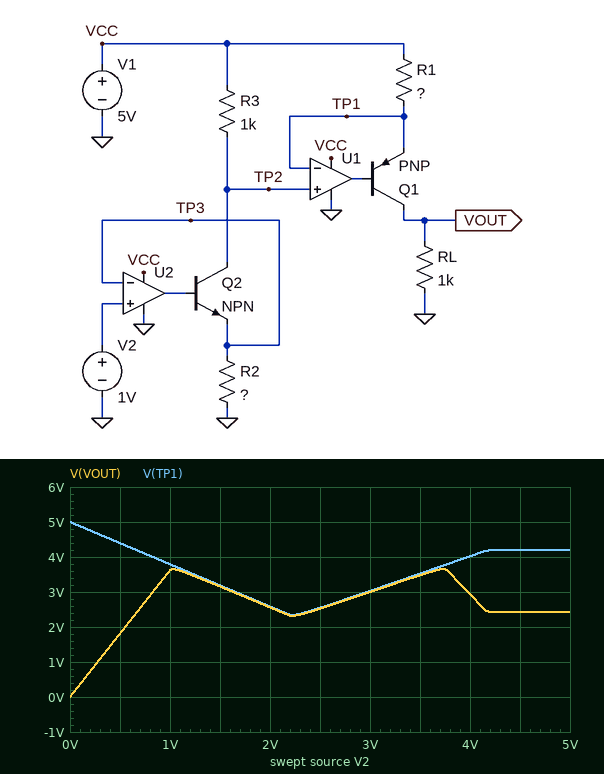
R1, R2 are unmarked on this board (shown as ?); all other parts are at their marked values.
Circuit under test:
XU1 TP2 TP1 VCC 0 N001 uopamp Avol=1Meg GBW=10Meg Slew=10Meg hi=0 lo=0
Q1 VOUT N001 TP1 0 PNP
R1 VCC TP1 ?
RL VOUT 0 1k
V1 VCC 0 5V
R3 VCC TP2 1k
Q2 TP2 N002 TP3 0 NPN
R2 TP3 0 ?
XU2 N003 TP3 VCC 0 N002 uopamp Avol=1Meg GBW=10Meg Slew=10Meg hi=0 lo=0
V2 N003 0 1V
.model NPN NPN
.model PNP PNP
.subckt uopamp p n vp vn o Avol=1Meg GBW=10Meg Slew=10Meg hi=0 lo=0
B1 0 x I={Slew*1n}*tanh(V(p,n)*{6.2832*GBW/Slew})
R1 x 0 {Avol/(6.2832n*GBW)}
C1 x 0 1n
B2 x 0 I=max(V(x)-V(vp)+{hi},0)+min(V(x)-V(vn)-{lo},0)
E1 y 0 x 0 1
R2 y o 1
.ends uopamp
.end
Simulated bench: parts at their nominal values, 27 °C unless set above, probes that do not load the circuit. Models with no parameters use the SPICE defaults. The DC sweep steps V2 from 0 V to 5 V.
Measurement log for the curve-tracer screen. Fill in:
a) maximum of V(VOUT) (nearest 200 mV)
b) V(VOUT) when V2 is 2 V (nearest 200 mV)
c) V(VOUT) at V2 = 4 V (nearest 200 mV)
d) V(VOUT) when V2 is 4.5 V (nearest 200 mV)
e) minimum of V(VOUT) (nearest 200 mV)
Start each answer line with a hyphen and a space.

- 3.6 V
- 2.6 V
- 3.0 V
- 2.4 V
- 0 V
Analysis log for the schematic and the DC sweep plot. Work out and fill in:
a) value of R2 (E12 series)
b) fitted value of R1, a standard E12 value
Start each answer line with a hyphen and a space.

- 820 Ω
- 330 Ω
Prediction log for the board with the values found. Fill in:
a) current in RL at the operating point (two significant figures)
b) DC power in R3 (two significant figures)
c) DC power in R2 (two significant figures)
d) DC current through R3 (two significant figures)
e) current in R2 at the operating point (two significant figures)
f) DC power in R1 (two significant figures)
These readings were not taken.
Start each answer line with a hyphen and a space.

- 3.6 mA
- 1.5 mW
- 1.2 mW
- 1.2 mA
- 1.2 mA
- 4.4 mW
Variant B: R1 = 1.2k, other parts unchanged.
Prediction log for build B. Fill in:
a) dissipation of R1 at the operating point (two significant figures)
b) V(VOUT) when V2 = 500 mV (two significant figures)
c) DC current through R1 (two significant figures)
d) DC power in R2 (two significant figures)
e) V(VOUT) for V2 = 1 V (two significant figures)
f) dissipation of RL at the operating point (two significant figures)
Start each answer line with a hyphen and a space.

- 1.2 mW
- 500 mV
- 1.0 mA
- 1.2 mW
- 1.0 V
- 990 µW
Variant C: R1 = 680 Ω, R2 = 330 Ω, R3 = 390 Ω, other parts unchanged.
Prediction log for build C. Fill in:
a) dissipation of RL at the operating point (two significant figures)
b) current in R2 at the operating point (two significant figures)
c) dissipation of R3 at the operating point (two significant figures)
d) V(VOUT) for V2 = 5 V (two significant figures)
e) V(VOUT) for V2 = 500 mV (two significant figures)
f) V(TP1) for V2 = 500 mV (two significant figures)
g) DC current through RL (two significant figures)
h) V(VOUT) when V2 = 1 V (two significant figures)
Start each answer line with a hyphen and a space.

- 2.9 mW
- 3.0 mA
- 3.5 mW
- 1.2 V
- 850 mV
- 4.4 V
- 1.7 mA
- 1.7 V
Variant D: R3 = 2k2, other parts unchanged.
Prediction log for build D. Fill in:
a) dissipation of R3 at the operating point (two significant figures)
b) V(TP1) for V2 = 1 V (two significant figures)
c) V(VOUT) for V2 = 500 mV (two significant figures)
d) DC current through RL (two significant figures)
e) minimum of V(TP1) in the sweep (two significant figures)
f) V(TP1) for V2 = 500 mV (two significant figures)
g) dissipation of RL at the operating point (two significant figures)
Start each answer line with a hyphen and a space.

- 3.2 mW
- 2.3 V
- 3.6 V
- 2.3 mA
- 1.5 V
- 3.7 V
- 5.4 mW
